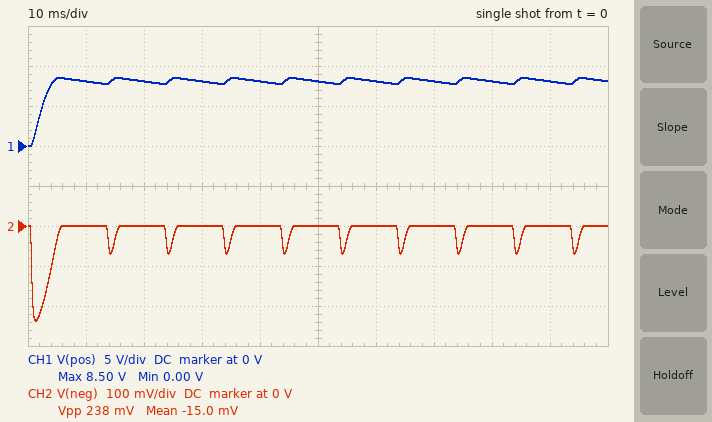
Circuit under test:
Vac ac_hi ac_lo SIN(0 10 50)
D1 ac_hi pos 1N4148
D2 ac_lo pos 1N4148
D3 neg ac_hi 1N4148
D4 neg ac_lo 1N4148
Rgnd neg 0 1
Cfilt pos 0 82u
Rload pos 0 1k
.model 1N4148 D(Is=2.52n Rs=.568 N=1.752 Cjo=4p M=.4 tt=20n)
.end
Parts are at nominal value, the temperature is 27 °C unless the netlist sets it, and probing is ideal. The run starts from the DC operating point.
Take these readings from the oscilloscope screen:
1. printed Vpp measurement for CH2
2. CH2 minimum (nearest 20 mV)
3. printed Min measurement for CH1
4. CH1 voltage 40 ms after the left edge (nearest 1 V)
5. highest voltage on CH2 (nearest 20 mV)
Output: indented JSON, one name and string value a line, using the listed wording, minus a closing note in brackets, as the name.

{
  "printed Vpp measurement for CH2": "238 mV",
  "CH2 minimum": "-240 mV",
  "printed Min measurement for CH1": "0.00 V",
  "CH1 voltage 40 ms after the left edge": "8 V",
  "highest voltage on CH2": "0 V"
}
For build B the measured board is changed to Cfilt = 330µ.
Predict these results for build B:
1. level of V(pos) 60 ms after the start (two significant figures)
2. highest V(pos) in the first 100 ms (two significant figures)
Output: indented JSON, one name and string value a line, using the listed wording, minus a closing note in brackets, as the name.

{
  "level of V(pos) 60 ms after the start": "8.3 V",
  "highest V(pos) in the first 100 ms": "8.4 V"
}
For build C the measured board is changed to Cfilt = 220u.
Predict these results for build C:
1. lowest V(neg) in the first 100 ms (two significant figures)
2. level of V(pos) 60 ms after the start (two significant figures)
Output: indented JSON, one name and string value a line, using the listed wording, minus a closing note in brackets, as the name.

{
  "lowest V(neg) in the first 100 ms": "-570 mV",
  "level of V(pos) 60 ms after the start": "8.2 V"
}
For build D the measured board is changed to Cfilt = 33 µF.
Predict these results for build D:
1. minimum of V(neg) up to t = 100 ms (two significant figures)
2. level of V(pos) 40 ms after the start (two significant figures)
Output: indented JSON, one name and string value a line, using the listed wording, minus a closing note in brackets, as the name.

{
  "minimum of V(neg) up to t = 100 ms": "-100 mV",
  "level of V(pos) 40 ms after the start": "7.5 V"
}
